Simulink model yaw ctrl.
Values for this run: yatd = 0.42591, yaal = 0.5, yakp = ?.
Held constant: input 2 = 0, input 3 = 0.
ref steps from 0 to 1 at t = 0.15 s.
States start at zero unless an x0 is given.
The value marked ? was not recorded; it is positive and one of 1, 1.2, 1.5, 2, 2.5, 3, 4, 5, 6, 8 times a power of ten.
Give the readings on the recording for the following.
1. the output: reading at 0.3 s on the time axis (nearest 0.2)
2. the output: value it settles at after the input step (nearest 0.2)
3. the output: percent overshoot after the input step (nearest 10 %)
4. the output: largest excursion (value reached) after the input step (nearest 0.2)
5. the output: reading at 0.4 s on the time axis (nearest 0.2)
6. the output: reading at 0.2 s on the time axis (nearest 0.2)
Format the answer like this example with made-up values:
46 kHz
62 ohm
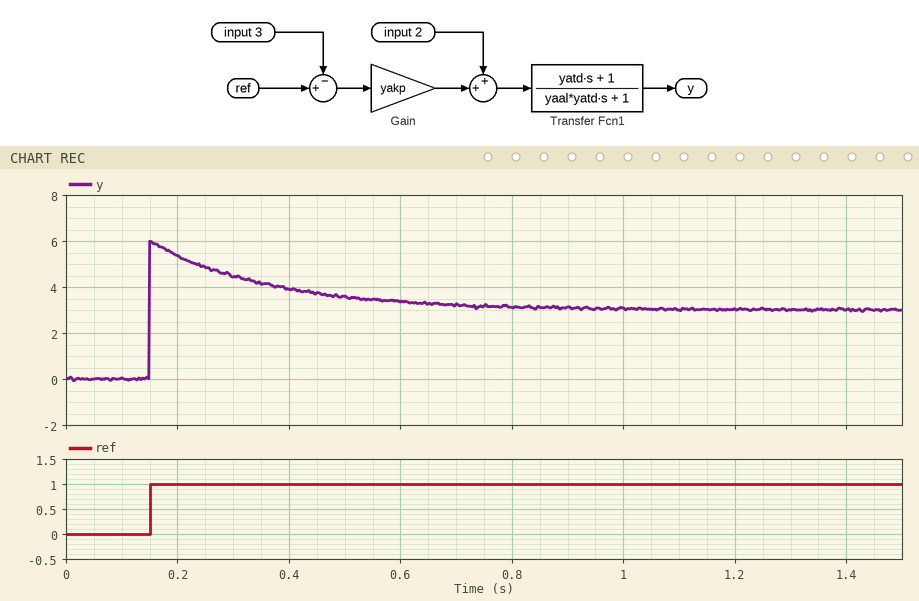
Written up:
4.4
3.0
100 %
6.0
4.0
5.4
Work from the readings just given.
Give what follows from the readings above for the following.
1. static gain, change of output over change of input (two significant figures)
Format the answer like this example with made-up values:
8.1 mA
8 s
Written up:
3.0
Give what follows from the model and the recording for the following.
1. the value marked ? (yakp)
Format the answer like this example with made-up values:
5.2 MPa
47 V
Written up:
3
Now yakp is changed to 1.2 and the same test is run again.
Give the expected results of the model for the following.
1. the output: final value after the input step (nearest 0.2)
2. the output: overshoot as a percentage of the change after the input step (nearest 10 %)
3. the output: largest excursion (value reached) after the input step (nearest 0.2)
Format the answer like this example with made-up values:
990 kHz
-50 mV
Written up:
1.2
100 %
2.4
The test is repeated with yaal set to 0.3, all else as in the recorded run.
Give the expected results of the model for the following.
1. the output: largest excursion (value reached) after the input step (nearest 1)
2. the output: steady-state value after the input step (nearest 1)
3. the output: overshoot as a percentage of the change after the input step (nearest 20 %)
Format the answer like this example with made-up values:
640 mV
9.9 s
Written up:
10
3
240 %
